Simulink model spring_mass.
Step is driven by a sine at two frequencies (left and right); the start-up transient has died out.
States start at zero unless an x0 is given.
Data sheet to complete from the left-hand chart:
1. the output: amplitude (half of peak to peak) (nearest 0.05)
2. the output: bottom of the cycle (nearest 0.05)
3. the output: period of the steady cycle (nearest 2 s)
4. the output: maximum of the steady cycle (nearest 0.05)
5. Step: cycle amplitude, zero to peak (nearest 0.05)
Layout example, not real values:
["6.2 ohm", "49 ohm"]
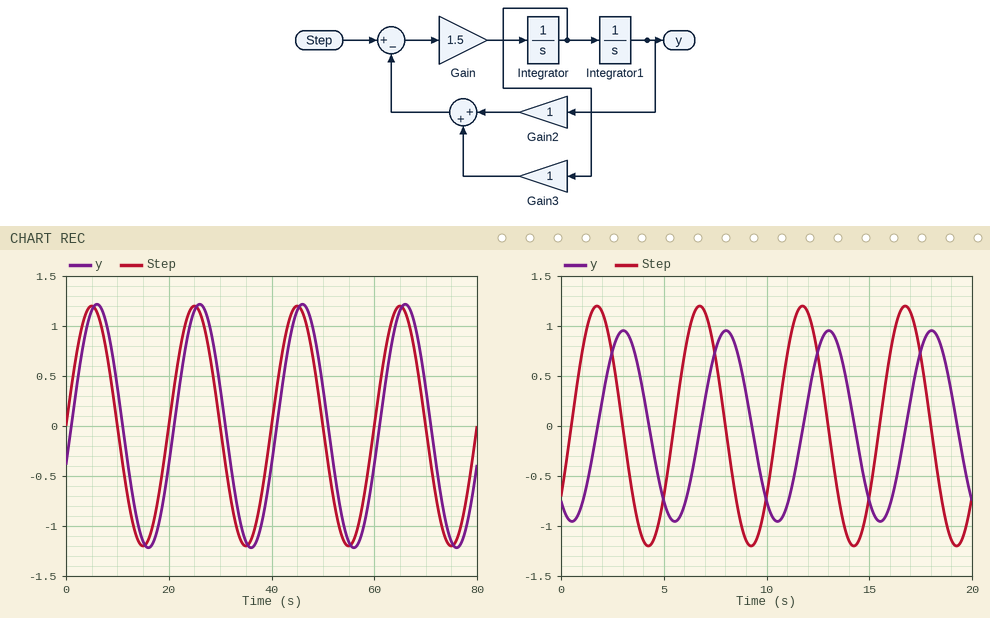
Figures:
["1.20", "-1.20", "20 s", "1.20", "1.20"]
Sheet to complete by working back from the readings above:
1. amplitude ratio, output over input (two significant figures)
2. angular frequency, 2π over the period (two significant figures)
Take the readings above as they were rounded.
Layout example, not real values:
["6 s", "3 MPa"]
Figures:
["1.0", "0.31 rad/s"]
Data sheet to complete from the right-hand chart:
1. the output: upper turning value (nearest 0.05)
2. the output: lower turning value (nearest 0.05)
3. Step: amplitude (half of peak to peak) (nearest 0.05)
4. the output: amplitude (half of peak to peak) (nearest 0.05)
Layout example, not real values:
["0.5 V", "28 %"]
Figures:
["0.95", "-0.95", "1.20", "0.95"]
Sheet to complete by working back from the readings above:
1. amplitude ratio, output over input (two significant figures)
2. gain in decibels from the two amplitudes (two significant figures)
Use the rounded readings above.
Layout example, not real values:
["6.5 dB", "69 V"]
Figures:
["0.79", "-2.0 dB"]
